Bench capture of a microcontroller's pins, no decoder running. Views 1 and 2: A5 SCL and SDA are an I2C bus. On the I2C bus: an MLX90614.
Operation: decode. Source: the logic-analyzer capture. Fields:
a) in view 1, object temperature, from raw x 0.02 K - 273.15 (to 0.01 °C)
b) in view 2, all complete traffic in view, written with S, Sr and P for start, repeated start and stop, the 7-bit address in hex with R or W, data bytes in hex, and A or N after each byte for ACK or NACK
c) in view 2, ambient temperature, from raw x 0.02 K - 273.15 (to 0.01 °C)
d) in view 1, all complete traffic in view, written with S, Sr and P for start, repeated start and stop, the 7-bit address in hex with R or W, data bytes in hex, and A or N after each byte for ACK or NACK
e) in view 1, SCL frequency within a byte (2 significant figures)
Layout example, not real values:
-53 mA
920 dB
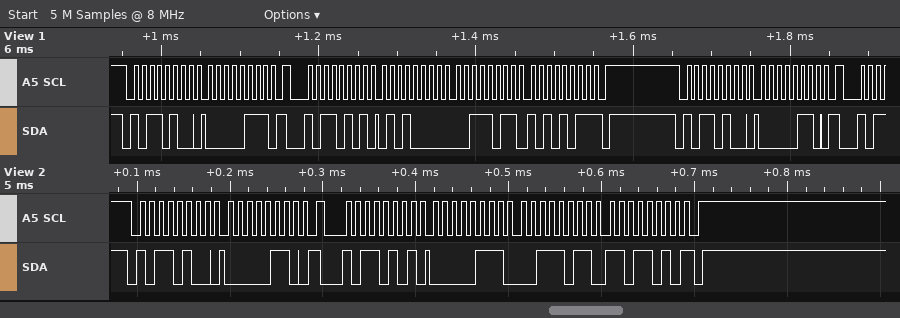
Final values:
30.53 °C
S 5AW A 06 A Sr 5AR A 07 A 3B A DA N P
29.07 °C
S 5AW A 07 A Sr 5AR A 50 A 3B A AB N P S 5AW A 06 A
100 kHz
